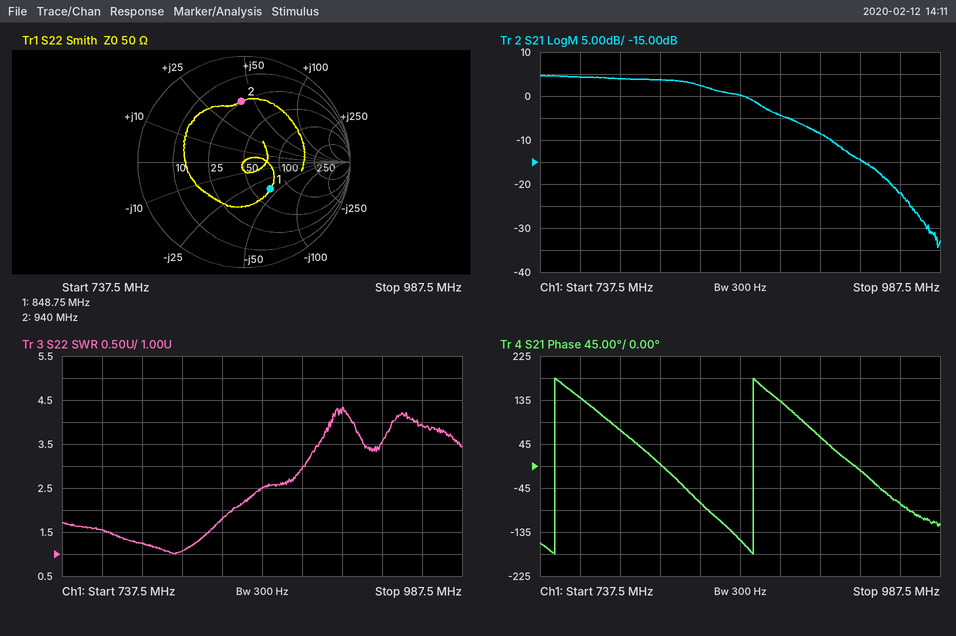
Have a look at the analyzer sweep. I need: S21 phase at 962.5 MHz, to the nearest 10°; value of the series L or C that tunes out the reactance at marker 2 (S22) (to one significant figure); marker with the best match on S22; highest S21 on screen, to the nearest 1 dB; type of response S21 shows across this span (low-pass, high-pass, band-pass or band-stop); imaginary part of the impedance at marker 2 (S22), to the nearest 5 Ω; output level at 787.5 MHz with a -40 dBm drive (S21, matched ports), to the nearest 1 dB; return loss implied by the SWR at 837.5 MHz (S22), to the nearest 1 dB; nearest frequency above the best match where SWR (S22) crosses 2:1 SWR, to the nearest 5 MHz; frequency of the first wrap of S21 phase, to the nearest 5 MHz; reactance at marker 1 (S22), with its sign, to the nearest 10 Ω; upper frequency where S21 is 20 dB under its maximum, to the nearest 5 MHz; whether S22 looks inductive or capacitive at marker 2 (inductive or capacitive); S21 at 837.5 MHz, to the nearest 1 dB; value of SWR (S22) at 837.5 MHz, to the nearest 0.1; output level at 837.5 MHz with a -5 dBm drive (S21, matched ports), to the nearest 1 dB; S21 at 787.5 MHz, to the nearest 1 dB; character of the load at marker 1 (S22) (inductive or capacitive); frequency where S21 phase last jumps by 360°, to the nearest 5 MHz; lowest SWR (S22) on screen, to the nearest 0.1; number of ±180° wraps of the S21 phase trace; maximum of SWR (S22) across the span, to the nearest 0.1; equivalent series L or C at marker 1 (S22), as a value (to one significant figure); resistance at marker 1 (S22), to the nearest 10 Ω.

-80°
4 pF
marker 1
5 dB
low-pass
+40 Ω
-36 dBm
11 dB
845 MHz
745 MHz
-40 Ω
940 MHz
inductive
2 dB
1.8
-3 dBm
4 dB
capacitive
870 MHz
1.0
2
4.3
5 pF
70 Ω
